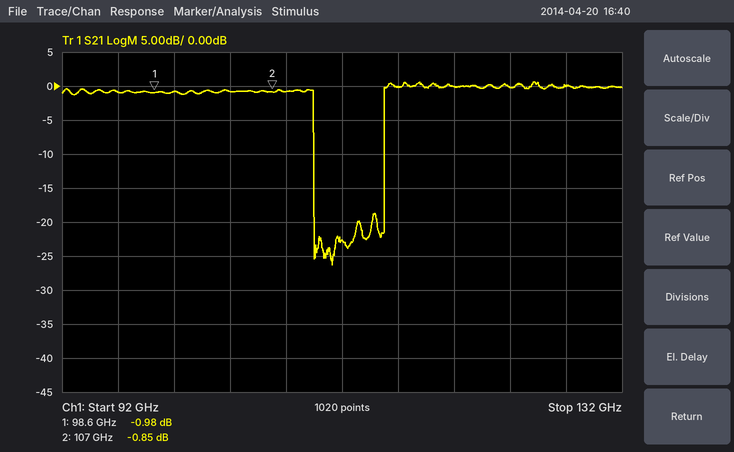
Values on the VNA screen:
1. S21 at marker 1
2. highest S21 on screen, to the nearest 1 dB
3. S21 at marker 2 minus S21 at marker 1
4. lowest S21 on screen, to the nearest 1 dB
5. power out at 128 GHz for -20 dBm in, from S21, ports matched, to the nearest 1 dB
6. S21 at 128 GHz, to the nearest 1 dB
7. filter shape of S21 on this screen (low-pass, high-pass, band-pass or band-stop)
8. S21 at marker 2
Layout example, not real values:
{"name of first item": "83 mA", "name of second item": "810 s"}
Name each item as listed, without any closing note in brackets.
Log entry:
{"S21 at marker 1": "-0.98 dB", "highest S21 on screen, to the nearest 1 dB": "1 dB", "S21 at marker 2 minus S21 at marker 1": "0.13 dB", "lowest S21 on screen, to the nearest 1 dB": "-26 dB", "power out at 128 GHz for -20 dBm in, from S21, ports matched, to the nearest 1 dB": "-20 dBm", "S21 at 128 GHz, to the nearest 1 dB": "0 dB", "filter shape of S21 on this screen": "band-stop", "S21 at marker 2": "-0.85 dB"}
